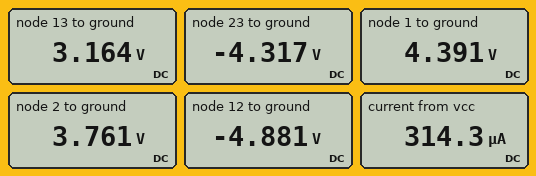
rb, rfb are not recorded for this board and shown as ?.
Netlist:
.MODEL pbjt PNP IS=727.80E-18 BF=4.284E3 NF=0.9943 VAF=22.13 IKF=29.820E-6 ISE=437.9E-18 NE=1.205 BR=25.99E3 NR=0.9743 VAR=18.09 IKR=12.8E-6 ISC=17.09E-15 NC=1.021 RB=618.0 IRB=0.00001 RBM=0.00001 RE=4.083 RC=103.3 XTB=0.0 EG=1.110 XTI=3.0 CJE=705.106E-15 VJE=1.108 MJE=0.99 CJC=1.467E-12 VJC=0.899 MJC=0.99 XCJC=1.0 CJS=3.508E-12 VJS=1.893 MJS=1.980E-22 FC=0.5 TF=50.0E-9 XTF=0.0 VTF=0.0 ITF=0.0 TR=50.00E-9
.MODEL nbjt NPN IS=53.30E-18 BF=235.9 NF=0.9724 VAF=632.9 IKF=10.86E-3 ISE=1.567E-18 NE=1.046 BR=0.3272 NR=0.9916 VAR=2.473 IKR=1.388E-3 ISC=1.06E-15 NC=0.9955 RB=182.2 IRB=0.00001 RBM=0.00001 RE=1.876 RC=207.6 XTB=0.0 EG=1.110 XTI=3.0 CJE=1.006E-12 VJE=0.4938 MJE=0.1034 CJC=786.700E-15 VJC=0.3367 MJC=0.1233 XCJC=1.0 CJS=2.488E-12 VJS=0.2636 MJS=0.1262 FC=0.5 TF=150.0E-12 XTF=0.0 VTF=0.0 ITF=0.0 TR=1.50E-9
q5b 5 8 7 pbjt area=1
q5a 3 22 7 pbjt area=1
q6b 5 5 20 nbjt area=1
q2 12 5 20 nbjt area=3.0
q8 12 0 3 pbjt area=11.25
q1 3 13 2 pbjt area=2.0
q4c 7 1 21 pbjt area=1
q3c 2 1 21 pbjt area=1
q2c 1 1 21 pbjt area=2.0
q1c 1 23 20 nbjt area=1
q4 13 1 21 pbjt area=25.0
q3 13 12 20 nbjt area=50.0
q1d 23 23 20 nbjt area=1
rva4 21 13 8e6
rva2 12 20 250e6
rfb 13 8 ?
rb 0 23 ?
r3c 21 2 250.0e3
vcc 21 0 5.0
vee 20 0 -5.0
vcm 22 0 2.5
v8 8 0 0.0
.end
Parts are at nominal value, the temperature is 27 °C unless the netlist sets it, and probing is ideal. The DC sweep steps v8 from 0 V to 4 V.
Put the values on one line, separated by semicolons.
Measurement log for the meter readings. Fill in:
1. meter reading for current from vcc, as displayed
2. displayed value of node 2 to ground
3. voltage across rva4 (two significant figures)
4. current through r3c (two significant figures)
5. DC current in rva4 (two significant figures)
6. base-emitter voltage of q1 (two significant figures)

314.3 µA; 3.761 V; 1.8 V; 5.0 µA; 230 nA; -600 mV
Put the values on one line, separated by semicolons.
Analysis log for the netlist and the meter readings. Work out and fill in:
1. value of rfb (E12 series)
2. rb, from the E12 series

12 kΩ; 180 kΩ
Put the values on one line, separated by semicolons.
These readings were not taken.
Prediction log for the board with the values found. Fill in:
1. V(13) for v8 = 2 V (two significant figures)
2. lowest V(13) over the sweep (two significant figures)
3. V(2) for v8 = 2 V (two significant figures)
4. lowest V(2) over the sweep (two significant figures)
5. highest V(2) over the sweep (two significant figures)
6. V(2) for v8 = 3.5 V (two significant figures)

4.4 V; -26 mV; 4.9 V; 610 mV; 4.9 V; 610 mV
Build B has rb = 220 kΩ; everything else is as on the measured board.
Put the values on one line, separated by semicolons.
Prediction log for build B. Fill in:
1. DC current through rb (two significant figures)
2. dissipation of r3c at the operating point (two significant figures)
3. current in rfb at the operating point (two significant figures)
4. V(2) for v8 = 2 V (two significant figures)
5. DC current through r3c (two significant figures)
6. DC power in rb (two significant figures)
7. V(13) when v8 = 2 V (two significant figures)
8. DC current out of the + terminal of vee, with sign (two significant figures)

20 µA; 12 µW; 220 µA; 4.9 V; 7.0 µA; 85 µW; 4.3 V; -64 µA
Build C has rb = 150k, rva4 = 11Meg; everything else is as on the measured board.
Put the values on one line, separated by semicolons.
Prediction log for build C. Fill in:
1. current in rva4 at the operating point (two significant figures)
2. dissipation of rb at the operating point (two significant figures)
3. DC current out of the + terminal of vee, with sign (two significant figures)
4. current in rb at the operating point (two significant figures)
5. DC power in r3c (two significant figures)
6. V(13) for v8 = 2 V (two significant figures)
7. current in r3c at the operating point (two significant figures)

120 nA; 120 µW; -86 µA; 29 µA; 2.0 µW; 4.6 V; 2.8 µA
